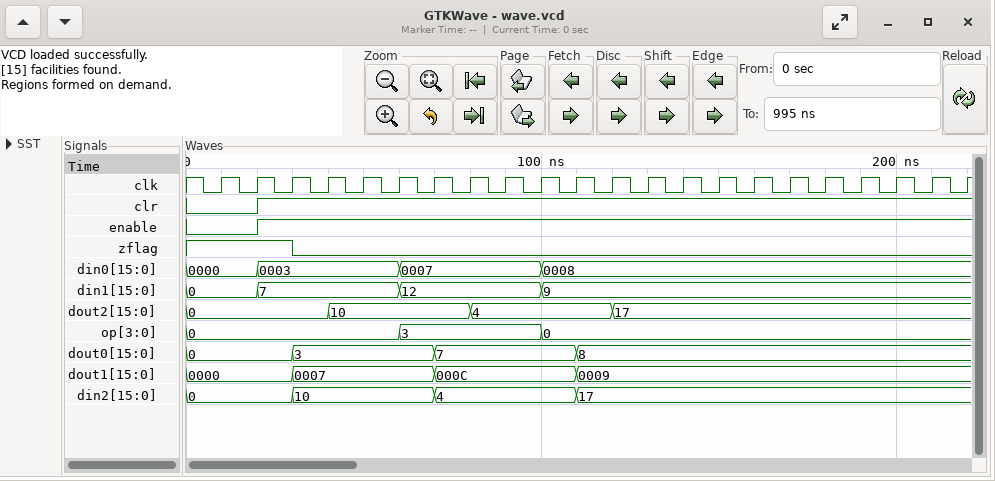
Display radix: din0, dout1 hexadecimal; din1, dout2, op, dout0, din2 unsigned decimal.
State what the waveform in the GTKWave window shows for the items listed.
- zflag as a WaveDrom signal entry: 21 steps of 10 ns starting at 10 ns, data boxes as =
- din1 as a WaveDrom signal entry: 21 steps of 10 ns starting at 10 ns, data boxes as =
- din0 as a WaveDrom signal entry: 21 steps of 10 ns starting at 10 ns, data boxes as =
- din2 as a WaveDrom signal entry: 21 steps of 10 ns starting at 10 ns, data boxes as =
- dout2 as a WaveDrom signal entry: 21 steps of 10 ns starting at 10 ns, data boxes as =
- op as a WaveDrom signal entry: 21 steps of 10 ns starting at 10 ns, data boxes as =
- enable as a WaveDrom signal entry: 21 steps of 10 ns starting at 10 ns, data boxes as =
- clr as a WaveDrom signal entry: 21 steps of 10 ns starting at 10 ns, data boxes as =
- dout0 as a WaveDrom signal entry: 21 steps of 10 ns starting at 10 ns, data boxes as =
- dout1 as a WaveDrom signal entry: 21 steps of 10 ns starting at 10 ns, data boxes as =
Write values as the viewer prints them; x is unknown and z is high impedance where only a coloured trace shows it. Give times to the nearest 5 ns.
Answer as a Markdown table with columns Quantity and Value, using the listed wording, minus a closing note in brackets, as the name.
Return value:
| Quantity | Value |
|---|---|
| zflag as a WaveDrom signal entry: 21 steps of 10 ns starting at 10 ns, data boxes as = | {name: 'zflag', wave: '1.0..................'} |
| din1 as a WaveDrom signal entry: 21 steps of 10 ns starting at 10 ns, data boxes as = | {name: 'din1', wave: '==...=...=...........', data: '0 7 12 9'} |
| din0 as a WaveDrom signal entry: 21 steps of 10 ns starting at 10 ns, data boxes as = | {name: 'din0', wave: '==...=...=...........', data: '0000 0003 0007 0008'} |
| din2 as a WaveDrom signal entry: 21 steps of 10 ns starting at 10 ns, data boxes as = | {name: 'din2', wave: '=.=...=...=..........', data: '0 10 4 17'} |
| dout2 as a WaveDrom signal entry: 21 steps of 10 ns starting at 10 ns, data boxes as = | {name: 'dout2', wave: '=..=...=...=.........', data: '0 10 4 17'} |
| op as a WaveDrom signal entry: 21 steps of 10 ns starting at 10 ns, data boxes as = | {name: 'op', wave: '=....=...=...........', data: '0 3 0'} |
| enable as a WaveDrom signal entry: 21 steps of 10 ns starting at 10 ns, data boxes as = | {name: 'enable', wave: '01...................'} |
| clr as a WaveDrom signal entry: 21 steps of 10 ns starting at 10 ns, data boxes as = | {name: 'clr', wave: '01...................'} |
| dout0 as a WaveDrom signal entry: 21 steps of 10 ns starting at 10 ns, data boxes as = | {name: 'dout0', wave: '=.=...=...=..........', data: '0 3 7 8'} |
| dout1 as a WaveDrom signal entry: 21 steps of 10 ns starting at 10 ns, data boxes as = | {name: 'dout1', wave: '=.=...=...=..........', data: '0000 0007 000C 0009'} |
